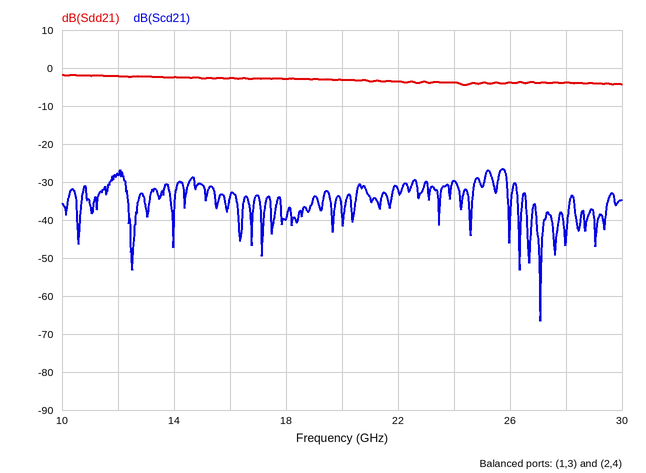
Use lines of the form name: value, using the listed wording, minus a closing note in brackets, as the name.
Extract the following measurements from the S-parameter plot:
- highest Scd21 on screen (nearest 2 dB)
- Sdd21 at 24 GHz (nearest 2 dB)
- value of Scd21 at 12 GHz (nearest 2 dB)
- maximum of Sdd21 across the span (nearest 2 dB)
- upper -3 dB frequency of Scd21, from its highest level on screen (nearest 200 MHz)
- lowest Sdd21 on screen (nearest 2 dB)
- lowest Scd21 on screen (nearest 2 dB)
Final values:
highest Scd21 on screen: -26 dB
Sdd21 at 24 GHz: -4 dB
value of Scd21 at 12 GHz: -28 dB
maximum of Sdd21 across the span: -2 dB
upper -3 dB frequency of Scd21, from its highest level on screen: 25.8 GHz
lowest Sdd21 on screen: -4 dB
lowest Scd21 on screen: -66 dB
